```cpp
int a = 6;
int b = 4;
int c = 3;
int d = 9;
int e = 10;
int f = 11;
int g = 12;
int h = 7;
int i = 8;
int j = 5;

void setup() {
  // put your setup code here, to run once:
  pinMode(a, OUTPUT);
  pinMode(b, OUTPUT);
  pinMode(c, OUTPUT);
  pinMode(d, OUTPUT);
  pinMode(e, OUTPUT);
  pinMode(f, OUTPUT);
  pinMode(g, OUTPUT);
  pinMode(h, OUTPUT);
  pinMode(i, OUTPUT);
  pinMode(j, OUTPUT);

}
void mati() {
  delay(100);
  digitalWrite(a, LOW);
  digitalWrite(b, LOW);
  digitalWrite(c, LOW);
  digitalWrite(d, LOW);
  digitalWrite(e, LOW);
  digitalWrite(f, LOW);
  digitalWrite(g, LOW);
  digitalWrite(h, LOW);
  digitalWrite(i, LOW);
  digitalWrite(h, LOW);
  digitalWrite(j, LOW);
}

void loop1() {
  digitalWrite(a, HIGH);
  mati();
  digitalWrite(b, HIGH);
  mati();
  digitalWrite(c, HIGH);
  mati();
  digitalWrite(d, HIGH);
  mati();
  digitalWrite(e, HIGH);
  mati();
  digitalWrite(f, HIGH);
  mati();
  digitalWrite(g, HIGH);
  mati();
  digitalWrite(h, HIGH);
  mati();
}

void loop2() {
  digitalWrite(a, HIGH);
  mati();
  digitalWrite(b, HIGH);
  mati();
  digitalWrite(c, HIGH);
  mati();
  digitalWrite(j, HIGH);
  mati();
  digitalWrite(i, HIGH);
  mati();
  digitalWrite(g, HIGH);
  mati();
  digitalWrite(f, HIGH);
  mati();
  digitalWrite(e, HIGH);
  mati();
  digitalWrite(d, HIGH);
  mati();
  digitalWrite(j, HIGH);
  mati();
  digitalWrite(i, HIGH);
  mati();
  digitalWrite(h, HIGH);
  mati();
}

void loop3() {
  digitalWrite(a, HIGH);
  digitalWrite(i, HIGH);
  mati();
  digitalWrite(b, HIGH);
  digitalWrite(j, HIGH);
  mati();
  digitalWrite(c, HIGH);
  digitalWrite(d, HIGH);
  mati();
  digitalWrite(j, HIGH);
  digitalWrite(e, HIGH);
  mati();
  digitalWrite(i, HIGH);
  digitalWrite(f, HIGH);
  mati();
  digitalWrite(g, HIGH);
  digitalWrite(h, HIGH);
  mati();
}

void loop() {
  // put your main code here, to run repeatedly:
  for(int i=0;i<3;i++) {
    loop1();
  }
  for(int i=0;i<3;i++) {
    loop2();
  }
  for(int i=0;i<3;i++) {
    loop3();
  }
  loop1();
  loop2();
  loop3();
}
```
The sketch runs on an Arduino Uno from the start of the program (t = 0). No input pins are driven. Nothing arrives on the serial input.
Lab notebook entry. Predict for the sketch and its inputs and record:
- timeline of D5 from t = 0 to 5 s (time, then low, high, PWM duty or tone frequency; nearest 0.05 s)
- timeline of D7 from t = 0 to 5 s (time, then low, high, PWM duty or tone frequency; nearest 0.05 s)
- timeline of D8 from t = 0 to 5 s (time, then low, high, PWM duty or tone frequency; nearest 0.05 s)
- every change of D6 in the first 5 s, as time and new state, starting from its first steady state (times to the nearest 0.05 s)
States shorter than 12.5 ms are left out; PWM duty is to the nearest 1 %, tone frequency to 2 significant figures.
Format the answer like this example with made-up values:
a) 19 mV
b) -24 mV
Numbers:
a) 0 s low; 2.7 s high; 2.8 s low; 3.3 s high; 3.4 s low; 3.9 s high; 4 s low; 4.5 s high; 4.6 s low
b) 0 s low; 0.7 s high; 0.8 s low; 1.5 s high; 1.6 s low; 2.3 s high; 2.4 s low; 3.5 s high; 3.6 s low; 4.7 s high; 4.8 s low
c) 0 s low; 2.8 s high; 2.9 s low; 3.4 s high; 3.5 s low; 4 s high; 4.1 s low; 4.6 s high; 4.7 s low
d) 0 s high; 0.1 s low; 0.8 s high; 0.9 s low; 1.6 s high; 1.7 s low; 2.4 s high; 2.5 s low; 3.6 s high; 3.7 s low; 4.8 s high; 4.9 s low
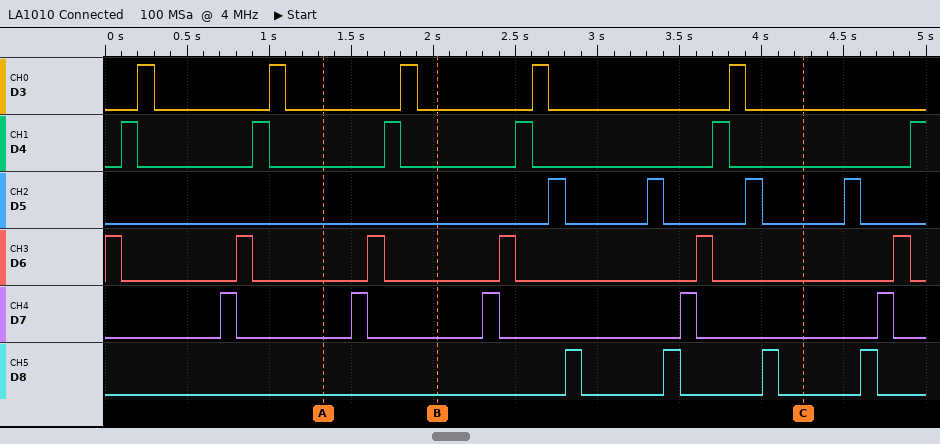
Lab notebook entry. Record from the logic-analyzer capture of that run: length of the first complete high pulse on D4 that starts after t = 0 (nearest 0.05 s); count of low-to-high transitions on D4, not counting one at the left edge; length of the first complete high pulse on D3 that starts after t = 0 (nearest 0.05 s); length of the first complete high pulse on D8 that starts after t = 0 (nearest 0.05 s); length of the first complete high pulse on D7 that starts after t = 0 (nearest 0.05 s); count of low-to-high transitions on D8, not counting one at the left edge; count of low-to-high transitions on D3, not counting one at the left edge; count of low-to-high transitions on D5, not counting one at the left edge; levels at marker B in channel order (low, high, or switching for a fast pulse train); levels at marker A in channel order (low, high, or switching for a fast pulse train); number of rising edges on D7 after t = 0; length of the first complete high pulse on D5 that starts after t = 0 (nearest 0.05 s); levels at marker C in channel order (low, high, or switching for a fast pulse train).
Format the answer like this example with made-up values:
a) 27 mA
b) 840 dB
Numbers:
a) 0.10 s
b) 6
c) 0.10 s
d) 0.10 s
e) 0.10 s
f) 4
g) 5
h) 4
i) D3 low, D4 low, D5 low, D6 low, D7 low, D8 low
j) D3 low, D4 low, D5 low, D6 low, D7 low, D8 low
k) 5
l) 0.10 s
m) D3 low, D4 low, D5 low, D6 low, D7 low, D8 low
